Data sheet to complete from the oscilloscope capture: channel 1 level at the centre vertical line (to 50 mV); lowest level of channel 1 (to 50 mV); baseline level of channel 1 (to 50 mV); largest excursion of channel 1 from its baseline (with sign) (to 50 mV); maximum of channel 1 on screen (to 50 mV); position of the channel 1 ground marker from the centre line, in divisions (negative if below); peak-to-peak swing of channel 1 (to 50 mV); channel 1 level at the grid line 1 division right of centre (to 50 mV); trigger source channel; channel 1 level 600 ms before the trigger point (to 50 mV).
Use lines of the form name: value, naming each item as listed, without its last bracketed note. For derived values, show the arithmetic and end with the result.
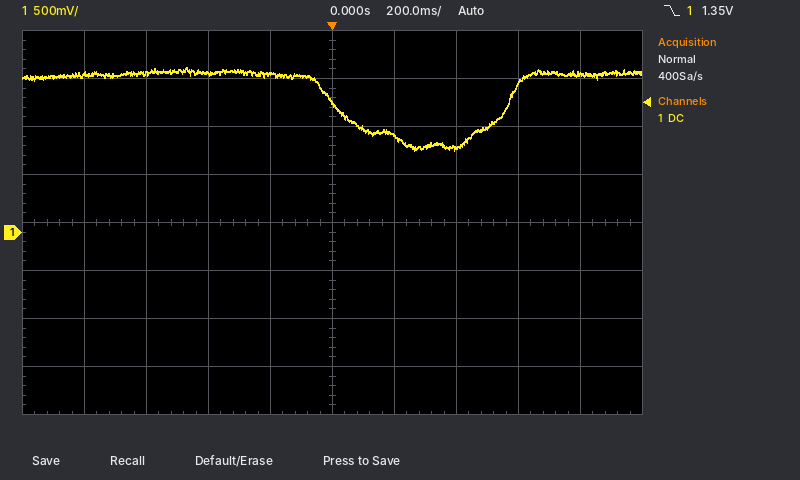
channel 1 level at the centre vertical line: 1.35 V
lowest level of channel 1: 850 mV
baseline level of channel 1: 1.65 V
largest excursion of channel 1 from its baseline (with sign): 850 mV − (1.65 V) = -800 mV
maximum of channel 1 on screen: 1.70 V
position of the channel 1 ground marker from the centre line, in divisions: -0.2 div
peak-to-peak swing of channel 1: 1.70 V − (850 mV) = 850 mV
channel 1 level at the grid line 1 division right of centre: 1.00 V
trigger source channel: channel 1
channel 1 level 600 ms before the trigger point: 1.65 V
